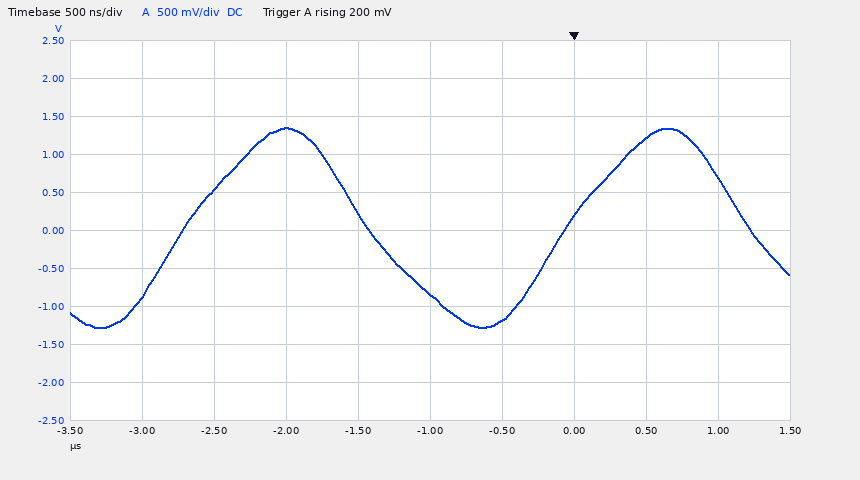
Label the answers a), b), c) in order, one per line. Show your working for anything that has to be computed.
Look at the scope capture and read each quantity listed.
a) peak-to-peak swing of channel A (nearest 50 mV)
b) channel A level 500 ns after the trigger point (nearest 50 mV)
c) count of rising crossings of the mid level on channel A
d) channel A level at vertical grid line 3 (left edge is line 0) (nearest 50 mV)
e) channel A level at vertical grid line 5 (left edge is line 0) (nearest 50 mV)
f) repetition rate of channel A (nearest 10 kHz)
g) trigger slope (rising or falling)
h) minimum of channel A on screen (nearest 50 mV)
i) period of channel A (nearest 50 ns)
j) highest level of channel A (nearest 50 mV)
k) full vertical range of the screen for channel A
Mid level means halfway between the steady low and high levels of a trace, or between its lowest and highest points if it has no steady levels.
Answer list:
a) 1.35 V − (-1.30 V) = 2.65 V
b) 1.20 V
c) 2
d) 1.35 V
e) -850 mV
f) 1 / 2.65 µs ≈ 377 kHz, so 380 kHz to the nearest 10 kHz
g) rising
h) -1.30 V
i) 2.65 µs
j) 1.35 V
k) 5 V
